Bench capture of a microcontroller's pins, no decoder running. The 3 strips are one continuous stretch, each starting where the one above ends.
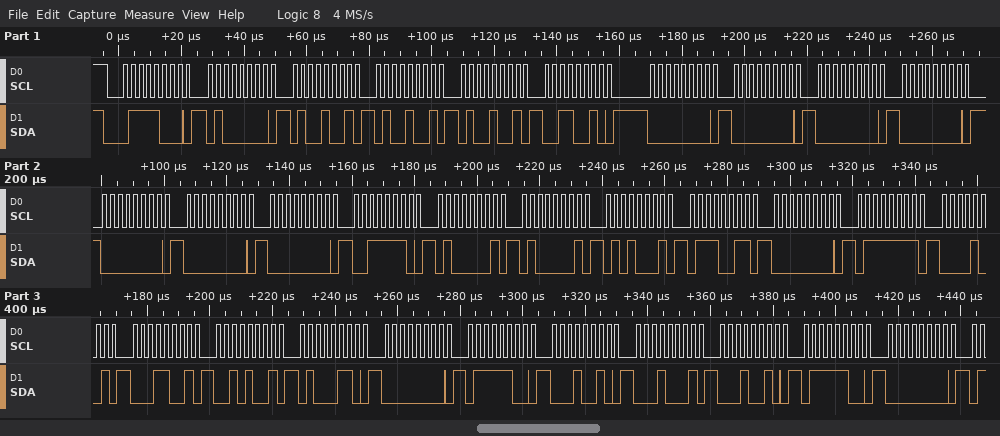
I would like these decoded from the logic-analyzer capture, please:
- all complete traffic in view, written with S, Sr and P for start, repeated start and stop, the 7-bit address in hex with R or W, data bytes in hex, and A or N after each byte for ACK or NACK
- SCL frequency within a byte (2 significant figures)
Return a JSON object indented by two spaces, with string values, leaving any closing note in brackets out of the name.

{
  "all complete traffic in view, written with S, Sr and P for start, repeated start and stop, the 7-bit address in hex with R or W, data bytes in hex, and A or N after each byte for ACK or NACK": "S 3CW A 40 A 49 A 49 A 49 A 32 A 00 A 00 A 00 A 00 A 00 A 00 A 00 A 3E A 41 A 41 A 51 A 73 A 00 A 7F A 09 A 19 A 29 A 46 A 00 A 7C A 12 A 11 A 12 A 7C A 00 A",
  "SCL frequency within a byte": "400 kHz"
}
